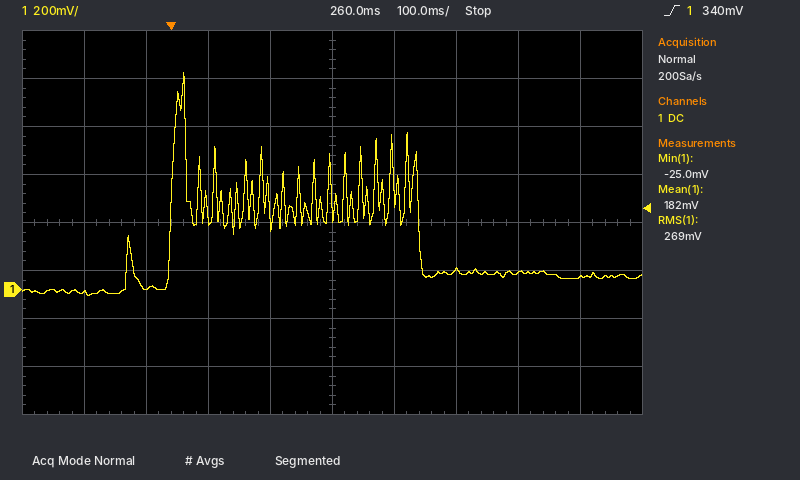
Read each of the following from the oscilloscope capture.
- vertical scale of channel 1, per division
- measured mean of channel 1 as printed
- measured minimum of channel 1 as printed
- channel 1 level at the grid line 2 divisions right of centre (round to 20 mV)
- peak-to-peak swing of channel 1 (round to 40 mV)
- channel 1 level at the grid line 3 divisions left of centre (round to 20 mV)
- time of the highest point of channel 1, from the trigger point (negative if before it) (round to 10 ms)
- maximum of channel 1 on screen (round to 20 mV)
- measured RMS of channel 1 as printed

200 mV
182 mV
-25.0 mV
80 mV
920 mV
0 mV
+20 ms
900 mV
269 mV
